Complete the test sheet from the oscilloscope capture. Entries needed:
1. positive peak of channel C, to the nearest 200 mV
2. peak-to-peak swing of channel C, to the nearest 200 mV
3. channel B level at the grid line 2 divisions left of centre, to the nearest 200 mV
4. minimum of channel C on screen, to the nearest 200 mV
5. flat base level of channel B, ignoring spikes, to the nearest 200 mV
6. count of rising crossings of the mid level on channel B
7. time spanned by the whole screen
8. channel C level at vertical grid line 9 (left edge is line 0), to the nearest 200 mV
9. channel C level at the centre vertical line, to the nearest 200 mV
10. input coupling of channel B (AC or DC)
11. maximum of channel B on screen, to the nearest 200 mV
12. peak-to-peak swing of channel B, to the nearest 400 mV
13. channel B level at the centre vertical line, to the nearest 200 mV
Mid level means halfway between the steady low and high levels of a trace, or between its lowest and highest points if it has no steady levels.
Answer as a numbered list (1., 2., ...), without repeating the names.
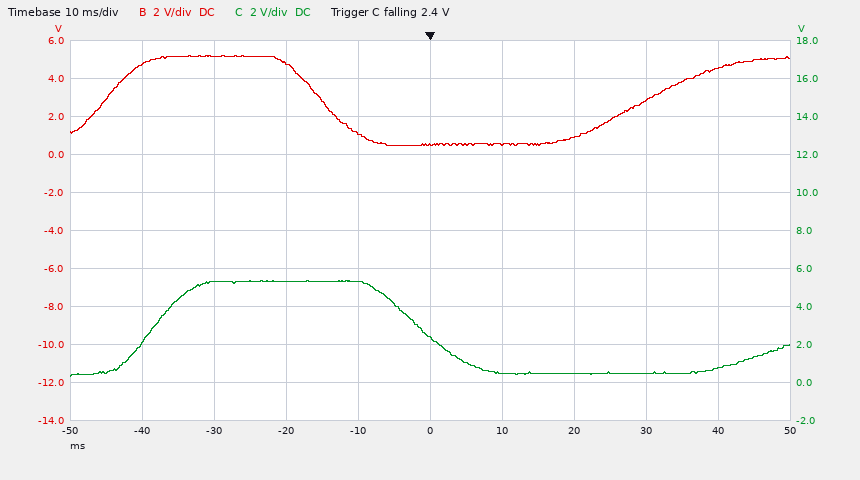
1. 5.4 V
2. 5.0 V
3. 4.8 V
4. 400 mV
5. 600 mV
6. 2
7. 100 ms
8. 800 mV
9. 2.4 V
10. DC
11. 5.2 V
12. 4.8 V
13. 600 mV
